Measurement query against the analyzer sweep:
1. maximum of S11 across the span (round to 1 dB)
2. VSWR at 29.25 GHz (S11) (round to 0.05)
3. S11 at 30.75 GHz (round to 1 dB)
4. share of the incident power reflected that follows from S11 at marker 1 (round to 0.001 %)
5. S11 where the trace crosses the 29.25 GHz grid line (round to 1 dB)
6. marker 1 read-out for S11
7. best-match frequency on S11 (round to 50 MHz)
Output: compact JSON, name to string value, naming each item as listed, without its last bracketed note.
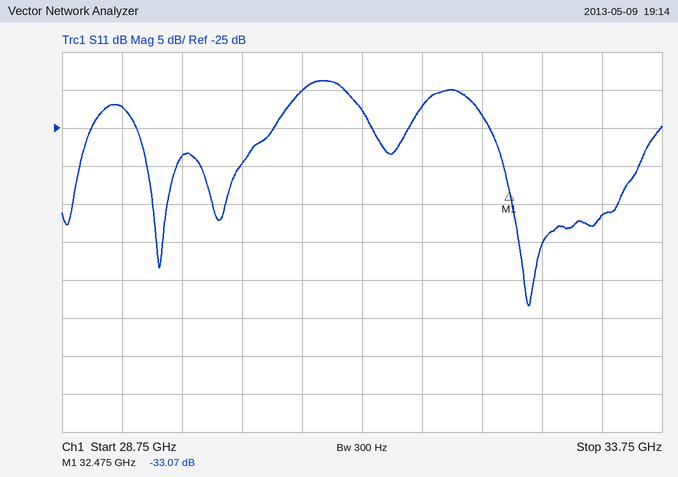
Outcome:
{"maximum of S11 across the span": "-19 dB", "VSWR at 29.25 GHz (S11)": "1.15", "S11 at 30.75 GHz": "-20 dB", "share of the incident power reflected that follows from S11 at marker 1": "0.049 %", "S11 where the trace crosses the 29.25 GHz grid line": "-22 dB", "marker 1 read-out for S11": "-33.07 dB", "best-match frequency on S11": "32.65 GHz"}
